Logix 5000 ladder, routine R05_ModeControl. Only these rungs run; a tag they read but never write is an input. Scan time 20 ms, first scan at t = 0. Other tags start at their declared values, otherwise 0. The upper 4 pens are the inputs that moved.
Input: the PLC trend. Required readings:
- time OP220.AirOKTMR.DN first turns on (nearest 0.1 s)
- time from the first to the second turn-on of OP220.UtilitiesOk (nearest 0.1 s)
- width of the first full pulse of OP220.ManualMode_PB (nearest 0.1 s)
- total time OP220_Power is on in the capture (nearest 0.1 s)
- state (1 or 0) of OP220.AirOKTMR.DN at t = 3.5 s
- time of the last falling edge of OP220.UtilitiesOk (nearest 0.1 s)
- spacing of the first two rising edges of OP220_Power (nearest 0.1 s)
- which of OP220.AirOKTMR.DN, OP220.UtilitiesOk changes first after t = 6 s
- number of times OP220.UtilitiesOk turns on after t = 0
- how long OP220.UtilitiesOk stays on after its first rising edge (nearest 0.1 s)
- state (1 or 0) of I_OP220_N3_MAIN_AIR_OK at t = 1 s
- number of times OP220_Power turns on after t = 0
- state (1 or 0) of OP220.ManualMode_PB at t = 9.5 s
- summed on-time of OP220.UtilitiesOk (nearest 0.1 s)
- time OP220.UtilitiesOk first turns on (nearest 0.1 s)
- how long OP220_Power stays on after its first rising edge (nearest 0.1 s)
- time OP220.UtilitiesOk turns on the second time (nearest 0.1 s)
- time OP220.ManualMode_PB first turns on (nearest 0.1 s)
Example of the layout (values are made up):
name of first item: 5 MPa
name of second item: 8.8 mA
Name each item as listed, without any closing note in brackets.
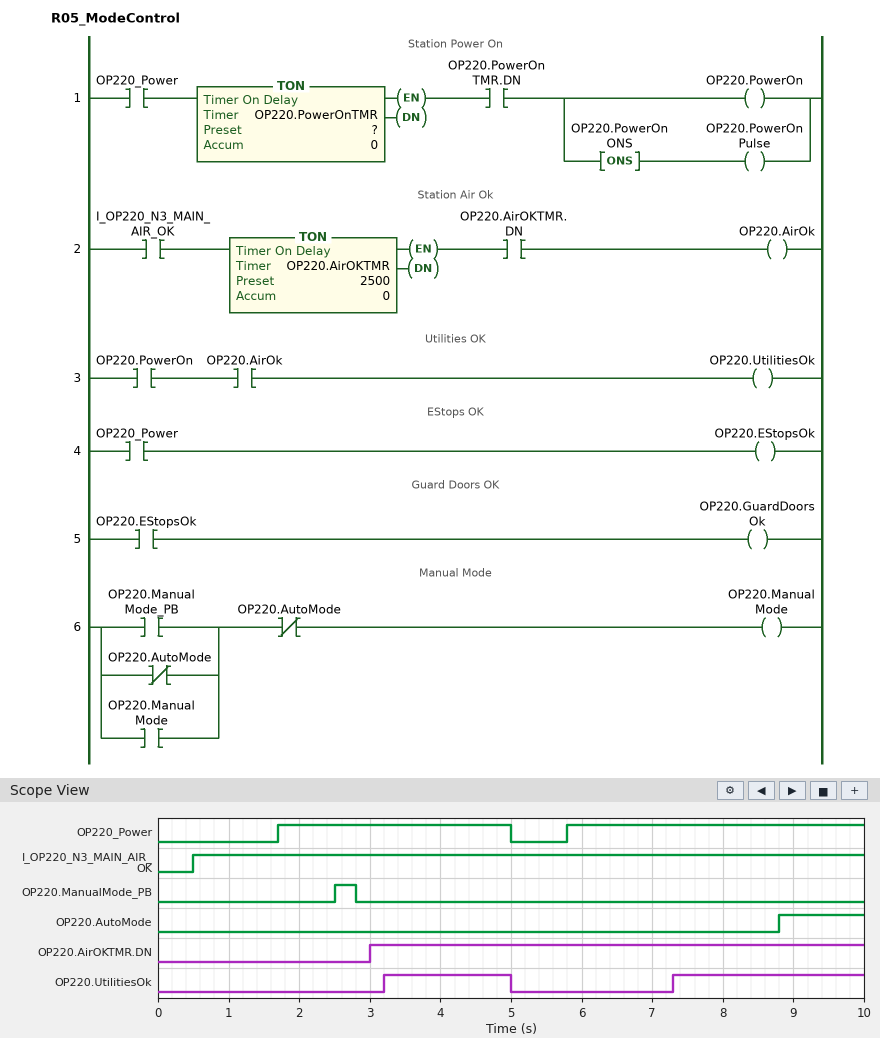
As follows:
time OP220.AirOKTMR.DN first turns on: 3.0 s
time from the first to the second turn-on of OP220.UtilitiesOk: 4.1 s
width of the first full pulse of OP220.ManualMode_PB: 0.3 s
total time OP220_Power is on in the capture: 7.5 s
state (1 or 0) of OP220.AirOKTMR.DN at t = 3.5 s: 1
time of the last falling edge of OP220.UtilitiesOk: 5.0 s
spacing of the first two rising edges of OP220_Power: 4.1 s
which of OP220.AirOKTMR.DN, OP220.UtilitiesOk changes first after t = 6 s: OP220.UtilitiesOk
number of times OP220.UtilitiesOk turns on after t = 0: 2
how long OP220.UtilitiesOk stays on after its first rising edge: 1.8 s
state (1 or 0) of I_OP220_N3_MAIN_AIR_OK at t = 1 s: 1
number of times OP220_Power turns on after t = 0: 2
state (1 or 0) of OP220.ManualMode_PB at t = 9.5 s: 0
summed on-time of OP220.UtilitiesOk: 4.5 s
time OP220.UtilitiesOk first turns on: 3.2 s
how long OP220_Power stays on after its first rising edge: 3.3 s
time OP220.UtilitiesOk turns on the second time: 7.3 s
time OP220.ManualMode_PB first turns on: 2.5 s
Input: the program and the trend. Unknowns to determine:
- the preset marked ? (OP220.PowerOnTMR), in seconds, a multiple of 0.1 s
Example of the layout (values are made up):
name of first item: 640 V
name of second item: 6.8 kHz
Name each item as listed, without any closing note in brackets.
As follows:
the preset marked ? (OP220.PowerOnTMR), in seconds, a multiple of 0.1 s: 1.5 s
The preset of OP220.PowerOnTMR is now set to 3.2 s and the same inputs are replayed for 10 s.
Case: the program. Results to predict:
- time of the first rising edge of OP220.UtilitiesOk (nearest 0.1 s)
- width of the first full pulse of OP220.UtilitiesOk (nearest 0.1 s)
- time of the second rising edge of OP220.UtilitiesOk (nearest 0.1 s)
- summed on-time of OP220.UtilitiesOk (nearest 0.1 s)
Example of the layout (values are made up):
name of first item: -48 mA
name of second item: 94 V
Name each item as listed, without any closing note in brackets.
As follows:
time of the first rising edge of OP220.UtilitiesOk: 4.9 s
width of the first full pulse of OP220.UtilitiesOk: 0.1 s
time of the second rising edge of OP220.UtilitiesOk: 9.0 s
summed on-time of OP220.UtilitiesOk: 1.1 s
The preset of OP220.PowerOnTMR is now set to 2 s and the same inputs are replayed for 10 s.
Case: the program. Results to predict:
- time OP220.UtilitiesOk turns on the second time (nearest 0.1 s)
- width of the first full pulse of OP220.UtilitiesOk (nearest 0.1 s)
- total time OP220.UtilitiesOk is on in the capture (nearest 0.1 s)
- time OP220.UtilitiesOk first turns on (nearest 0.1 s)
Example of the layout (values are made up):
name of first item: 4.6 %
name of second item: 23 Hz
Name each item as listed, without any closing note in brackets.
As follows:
time OP220.UtilitiesOk turns on the second time: 7.8 s
width of the first full pulse of OP220.UtilitiesOk: 1.3 s
total time OP220.UtilitiesOk is on in the capture: 3.5 s
time OP220.UtilitiesOk first turns on: 3.7 s
